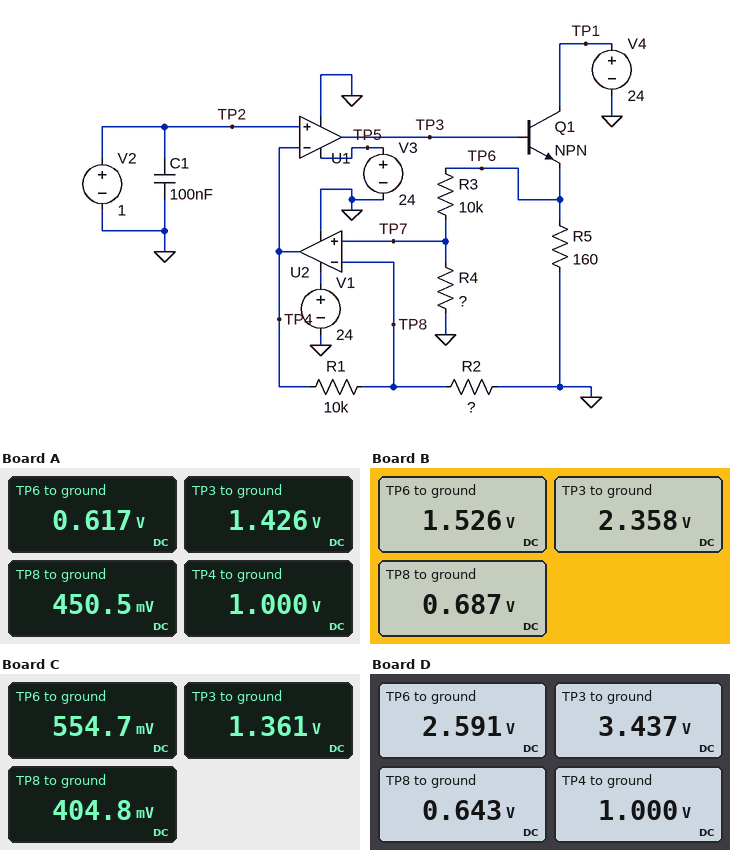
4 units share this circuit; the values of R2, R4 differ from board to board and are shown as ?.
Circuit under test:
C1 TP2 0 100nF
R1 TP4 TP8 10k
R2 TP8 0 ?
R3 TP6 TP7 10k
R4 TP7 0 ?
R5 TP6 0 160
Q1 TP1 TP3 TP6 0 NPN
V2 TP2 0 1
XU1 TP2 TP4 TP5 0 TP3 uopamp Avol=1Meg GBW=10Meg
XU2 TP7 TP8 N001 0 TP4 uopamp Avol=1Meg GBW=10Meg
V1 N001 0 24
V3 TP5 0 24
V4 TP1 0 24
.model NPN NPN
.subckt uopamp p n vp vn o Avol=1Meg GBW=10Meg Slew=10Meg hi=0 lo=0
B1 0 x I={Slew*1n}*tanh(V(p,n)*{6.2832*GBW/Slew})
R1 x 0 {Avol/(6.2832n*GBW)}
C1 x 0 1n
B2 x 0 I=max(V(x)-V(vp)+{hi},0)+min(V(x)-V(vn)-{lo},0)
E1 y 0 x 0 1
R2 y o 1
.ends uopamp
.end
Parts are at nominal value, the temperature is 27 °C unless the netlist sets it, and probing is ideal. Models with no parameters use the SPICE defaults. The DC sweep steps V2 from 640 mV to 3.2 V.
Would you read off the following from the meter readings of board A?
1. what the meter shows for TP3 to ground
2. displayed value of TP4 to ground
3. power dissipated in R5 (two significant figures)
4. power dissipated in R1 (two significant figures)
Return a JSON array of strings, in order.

["1.426 V", "1.000 V", "2.4 mW", "30 µW"]
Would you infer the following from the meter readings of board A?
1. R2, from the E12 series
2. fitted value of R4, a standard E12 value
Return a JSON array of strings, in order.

["8.2 kΩ", "27 kΩ"]
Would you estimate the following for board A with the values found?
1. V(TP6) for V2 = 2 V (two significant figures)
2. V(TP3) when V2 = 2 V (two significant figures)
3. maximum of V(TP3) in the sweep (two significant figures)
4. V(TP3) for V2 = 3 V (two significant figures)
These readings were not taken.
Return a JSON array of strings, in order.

["1.2 V", "2.1 V", "2.8 V", "2.7 V"]
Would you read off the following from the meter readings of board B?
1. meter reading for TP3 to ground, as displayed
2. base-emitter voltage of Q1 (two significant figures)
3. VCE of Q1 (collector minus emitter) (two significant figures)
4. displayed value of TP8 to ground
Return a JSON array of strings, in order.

["2.358 V", "830 mV", "22 V", "0.687 V"]
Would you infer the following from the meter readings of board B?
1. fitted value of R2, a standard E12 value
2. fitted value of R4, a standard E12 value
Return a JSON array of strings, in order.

["22 kΩ", "8.2 kΩ"]
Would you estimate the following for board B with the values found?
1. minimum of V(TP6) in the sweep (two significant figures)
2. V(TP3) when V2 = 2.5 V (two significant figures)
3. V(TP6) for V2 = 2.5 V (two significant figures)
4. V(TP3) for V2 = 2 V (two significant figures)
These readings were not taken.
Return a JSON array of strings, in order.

["980 mV", "4.7 V", "3.8 V", "3.9 V"]
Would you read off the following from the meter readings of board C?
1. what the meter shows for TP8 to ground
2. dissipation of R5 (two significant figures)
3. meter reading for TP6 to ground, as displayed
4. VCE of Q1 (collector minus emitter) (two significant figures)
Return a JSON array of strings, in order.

["404.8 mV", "1.9 mW", "554.7 mV", "23 V"]
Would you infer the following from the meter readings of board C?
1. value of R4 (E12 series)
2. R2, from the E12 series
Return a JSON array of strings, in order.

["27 kΩ", "6.8 kΩ"]
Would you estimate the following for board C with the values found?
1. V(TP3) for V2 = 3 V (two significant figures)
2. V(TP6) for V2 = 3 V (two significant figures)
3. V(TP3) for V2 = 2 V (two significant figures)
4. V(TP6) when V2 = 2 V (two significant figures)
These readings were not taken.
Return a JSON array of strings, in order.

["2.5 V", "1.7 V", "1.9 V", "1.1 V"]
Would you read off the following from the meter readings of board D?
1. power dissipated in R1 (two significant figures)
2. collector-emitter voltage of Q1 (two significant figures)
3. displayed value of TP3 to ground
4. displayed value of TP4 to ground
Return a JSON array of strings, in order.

["13 µW", "21 V", "3.437 V", "1.000 V"]
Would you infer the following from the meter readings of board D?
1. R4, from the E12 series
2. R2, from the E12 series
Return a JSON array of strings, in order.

["3.3 kΩ", "18 kΩ"]
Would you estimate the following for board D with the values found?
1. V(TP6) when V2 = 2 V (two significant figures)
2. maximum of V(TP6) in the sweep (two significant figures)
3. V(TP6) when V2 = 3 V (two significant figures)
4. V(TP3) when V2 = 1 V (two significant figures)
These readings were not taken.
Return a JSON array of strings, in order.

["5.2 V", "8.3 V", "7.8 V", "3.4 V"]
